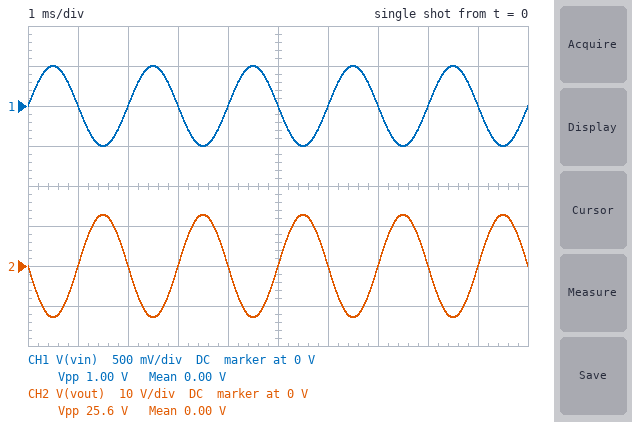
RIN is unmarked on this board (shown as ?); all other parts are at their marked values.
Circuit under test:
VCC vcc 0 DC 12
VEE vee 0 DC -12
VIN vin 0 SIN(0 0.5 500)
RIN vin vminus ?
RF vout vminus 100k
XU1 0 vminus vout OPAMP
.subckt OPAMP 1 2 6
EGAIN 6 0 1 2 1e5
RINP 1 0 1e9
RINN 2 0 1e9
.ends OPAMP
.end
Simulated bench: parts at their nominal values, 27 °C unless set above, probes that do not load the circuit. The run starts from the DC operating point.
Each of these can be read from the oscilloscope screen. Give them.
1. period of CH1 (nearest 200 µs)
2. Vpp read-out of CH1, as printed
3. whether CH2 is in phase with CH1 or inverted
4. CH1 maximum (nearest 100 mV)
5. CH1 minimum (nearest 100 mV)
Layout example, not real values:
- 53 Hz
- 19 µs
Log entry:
- 2.0 ms
- 1.00 V
- inverted
- 500 mV
- -500 mV
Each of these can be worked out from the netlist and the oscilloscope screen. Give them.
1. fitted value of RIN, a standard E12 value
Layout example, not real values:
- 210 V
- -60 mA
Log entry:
- 3.9 kΩ
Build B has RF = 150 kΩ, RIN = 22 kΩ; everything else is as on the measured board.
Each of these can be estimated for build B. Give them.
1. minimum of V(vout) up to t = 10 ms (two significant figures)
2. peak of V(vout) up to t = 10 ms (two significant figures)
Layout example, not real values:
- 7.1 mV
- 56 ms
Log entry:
- -3.4 V
- 3.4 V
